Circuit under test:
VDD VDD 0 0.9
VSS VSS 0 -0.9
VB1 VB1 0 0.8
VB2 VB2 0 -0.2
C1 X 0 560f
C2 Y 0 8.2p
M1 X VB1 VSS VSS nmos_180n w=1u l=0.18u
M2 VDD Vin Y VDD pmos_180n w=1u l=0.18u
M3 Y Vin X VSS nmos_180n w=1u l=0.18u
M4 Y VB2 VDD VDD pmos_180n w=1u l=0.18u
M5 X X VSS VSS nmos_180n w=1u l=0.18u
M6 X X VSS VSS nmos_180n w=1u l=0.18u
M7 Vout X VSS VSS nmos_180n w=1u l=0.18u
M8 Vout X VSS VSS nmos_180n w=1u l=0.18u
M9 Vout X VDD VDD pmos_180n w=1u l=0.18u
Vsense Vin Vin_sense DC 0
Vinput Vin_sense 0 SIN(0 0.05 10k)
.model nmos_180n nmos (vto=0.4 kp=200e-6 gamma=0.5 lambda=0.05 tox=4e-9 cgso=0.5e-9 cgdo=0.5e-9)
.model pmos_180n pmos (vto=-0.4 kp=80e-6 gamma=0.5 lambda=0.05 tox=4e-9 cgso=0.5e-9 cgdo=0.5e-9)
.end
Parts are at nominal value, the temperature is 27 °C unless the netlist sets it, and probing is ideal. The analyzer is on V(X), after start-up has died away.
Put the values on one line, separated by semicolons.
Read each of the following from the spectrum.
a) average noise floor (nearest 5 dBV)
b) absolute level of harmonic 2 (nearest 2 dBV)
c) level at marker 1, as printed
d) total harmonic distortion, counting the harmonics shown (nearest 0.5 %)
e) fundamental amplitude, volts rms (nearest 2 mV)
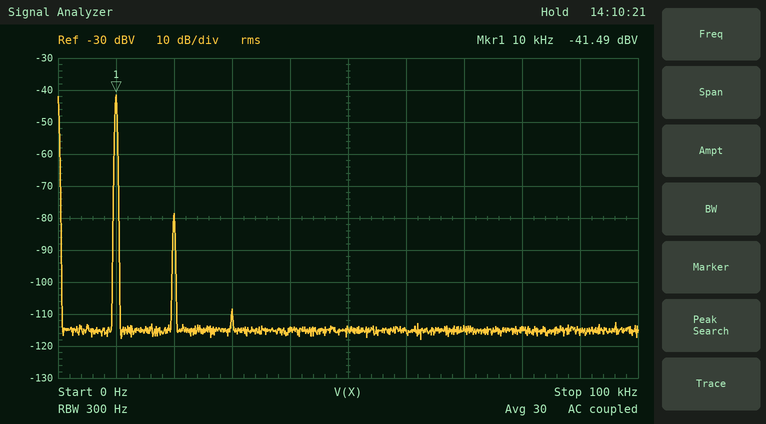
-115 dBV; -78 dBV; -41.49 dBV; 1.5 %; 8 mV
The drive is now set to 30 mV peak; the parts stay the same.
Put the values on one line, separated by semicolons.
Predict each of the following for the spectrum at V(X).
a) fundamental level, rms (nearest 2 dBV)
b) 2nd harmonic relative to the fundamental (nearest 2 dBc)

-46 dBV; -42 dBc
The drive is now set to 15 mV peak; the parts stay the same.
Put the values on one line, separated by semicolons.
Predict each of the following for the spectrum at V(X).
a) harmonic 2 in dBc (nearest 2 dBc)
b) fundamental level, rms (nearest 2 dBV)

-48 dBc; -52 dBV
